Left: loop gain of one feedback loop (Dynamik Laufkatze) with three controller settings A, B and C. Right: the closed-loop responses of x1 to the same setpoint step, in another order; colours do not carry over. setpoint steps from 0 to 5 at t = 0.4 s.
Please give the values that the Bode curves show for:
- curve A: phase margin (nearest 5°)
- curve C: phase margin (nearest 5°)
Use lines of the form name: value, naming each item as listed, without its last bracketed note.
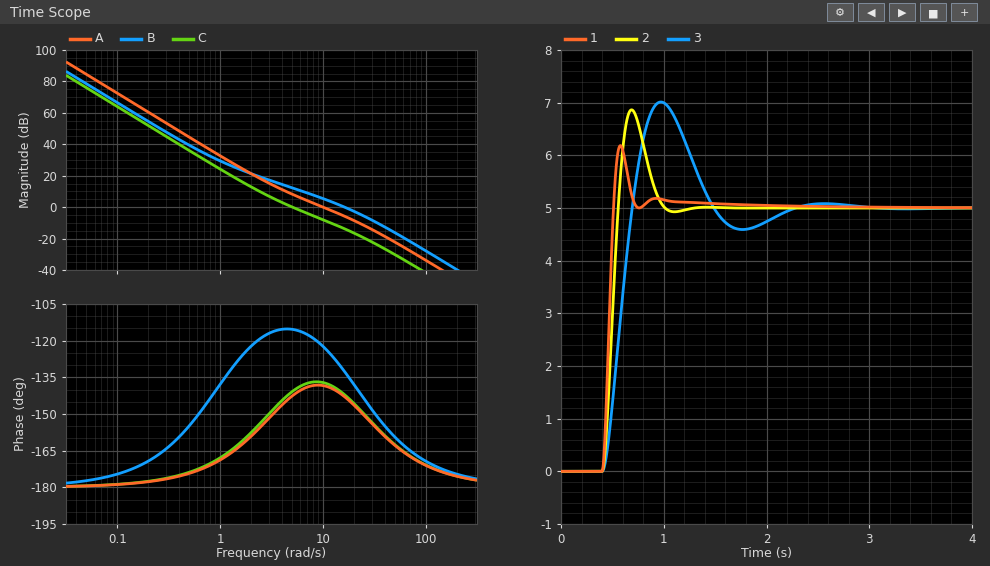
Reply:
curve A: phase margin: 40°
curve C: phase margin: 40°
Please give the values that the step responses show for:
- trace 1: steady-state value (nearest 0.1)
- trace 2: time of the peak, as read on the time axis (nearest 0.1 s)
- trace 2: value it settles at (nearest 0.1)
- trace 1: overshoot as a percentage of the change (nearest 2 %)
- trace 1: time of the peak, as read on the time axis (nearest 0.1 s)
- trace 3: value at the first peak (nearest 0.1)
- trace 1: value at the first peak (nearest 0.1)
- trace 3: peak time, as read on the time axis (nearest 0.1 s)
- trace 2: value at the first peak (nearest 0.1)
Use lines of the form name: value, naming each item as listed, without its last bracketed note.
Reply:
trace 1: steady-state value: 5.0
trace 2: time of the peak, as read on the time axis: 0.7 s
trace 2: value it settles at: 5.0
trace 1: overshoot as a percentage of the change: 24 %
trace 1: time of the peak, as read on the time axis: 0.6 s
trace 3: value at the first peak: 7.0
trace 1: value at the first peak: 6.2
trace 3: peak time, as read on the time axis: 1.0 s
trace 2: value at the first peak: 6.9
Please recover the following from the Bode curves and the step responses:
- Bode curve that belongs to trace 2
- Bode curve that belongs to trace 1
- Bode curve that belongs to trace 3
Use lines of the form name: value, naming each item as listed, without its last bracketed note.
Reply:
Bode curve that belongs to trace 2: A
Bode curve that belongs to trace 1: B
Bode curve that belongs to trace 3: C
